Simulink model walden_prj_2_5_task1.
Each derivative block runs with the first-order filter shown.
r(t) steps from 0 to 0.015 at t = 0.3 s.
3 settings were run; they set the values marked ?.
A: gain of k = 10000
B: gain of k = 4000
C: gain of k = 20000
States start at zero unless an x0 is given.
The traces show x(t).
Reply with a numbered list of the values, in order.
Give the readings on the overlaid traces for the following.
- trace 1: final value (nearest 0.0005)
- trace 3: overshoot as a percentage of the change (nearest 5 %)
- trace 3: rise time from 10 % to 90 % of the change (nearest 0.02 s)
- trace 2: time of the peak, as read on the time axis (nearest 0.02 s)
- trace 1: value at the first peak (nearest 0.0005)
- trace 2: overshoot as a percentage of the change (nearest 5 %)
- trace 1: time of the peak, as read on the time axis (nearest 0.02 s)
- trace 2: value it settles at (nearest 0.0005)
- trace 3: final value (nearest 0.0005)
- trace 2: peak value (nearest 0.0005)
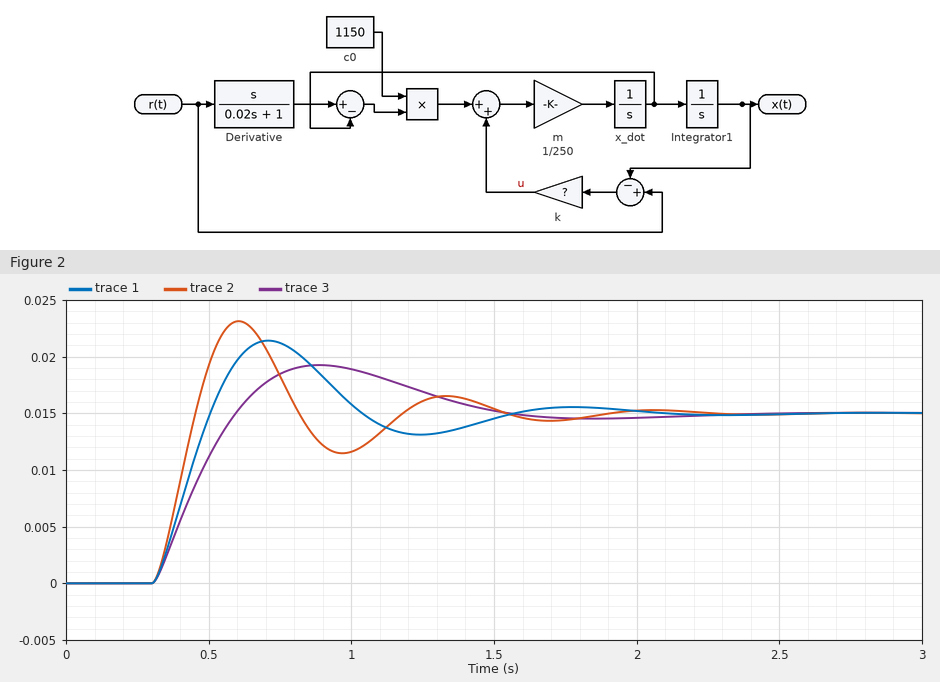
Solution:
1. 0.0150
2. 30 %
3. 0.22 s
4. 0.60 s
5. 0.0215
6. 55 %
7. 0.70 s
8. 0.0150
9. 0.0150
10. 0.0230
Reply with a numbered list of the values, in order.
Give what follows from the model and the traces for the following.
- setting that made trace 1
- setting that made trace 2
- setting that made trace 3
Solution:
1. A
2. C
3. B
